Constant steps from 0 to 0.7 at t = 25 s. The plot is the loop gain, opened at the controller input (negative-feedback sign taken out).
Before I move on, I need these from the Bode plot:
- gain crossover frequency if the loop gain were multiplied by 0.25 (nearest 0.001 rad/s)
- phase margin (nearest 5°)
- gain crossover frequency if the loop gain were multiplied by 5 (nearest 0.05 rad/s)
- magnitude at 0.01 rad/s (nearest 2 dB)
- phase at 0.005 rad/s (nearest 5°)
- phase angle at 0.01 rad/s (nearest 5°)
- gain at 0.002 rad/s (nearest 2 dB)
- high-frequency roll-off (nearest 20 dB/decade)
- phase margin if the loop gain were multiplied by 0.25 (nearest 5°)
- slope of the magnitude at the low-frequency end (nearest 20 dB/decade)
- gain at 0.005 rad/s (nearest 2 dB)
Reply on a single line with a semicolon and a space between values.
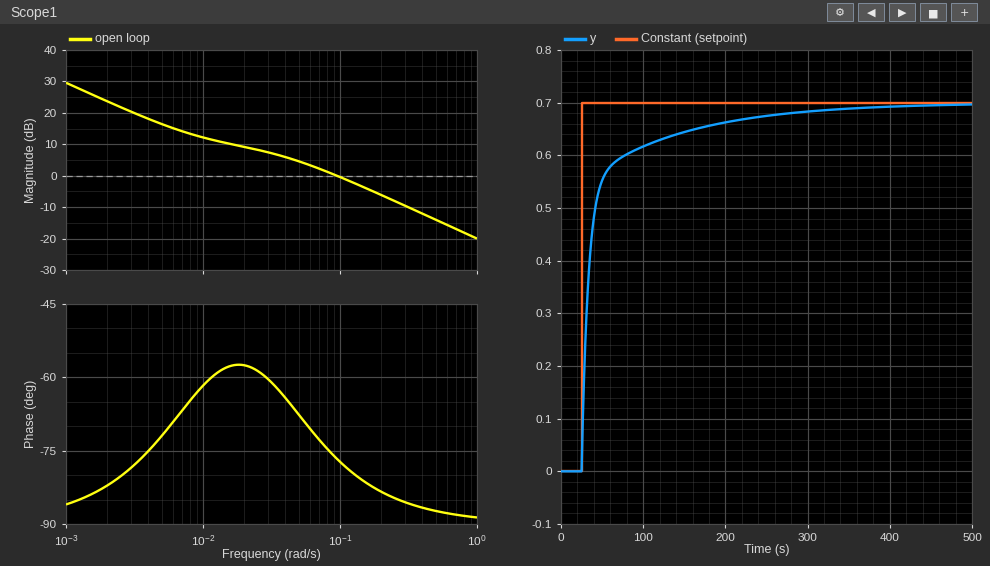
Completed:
0.010 rad/s; 105°; 0.50 rad/s; 12 dB; -70°; -60°; 24 dB; -20 dB/decade; 120°; -20 dB/decade; 16 dB
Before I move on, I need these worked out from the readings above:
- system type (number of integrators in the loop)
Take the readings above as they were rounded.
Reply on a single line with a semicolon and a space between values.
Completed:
1
